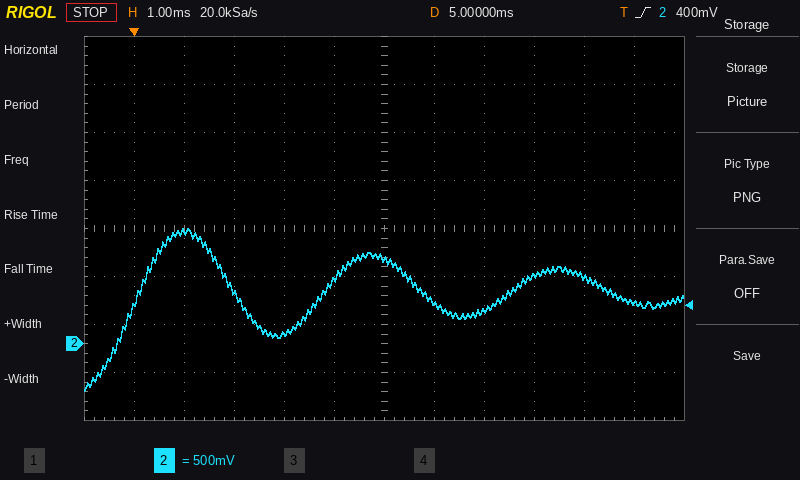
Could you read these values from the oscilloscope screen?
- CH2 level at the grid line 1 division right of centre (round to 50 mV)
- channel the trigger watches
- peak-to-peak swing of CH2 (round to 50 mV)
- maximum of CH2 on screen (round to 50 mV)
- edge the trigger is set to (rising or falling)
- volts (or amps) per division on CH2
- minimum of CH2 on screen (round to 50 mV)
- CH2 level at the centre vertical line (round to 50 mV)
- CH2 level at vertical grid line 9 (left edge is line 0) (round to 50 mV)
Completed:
450 mV
CH2
1.70 V
1.20 V
rising
500 mV
-500 mV
900 mV
700 mV
